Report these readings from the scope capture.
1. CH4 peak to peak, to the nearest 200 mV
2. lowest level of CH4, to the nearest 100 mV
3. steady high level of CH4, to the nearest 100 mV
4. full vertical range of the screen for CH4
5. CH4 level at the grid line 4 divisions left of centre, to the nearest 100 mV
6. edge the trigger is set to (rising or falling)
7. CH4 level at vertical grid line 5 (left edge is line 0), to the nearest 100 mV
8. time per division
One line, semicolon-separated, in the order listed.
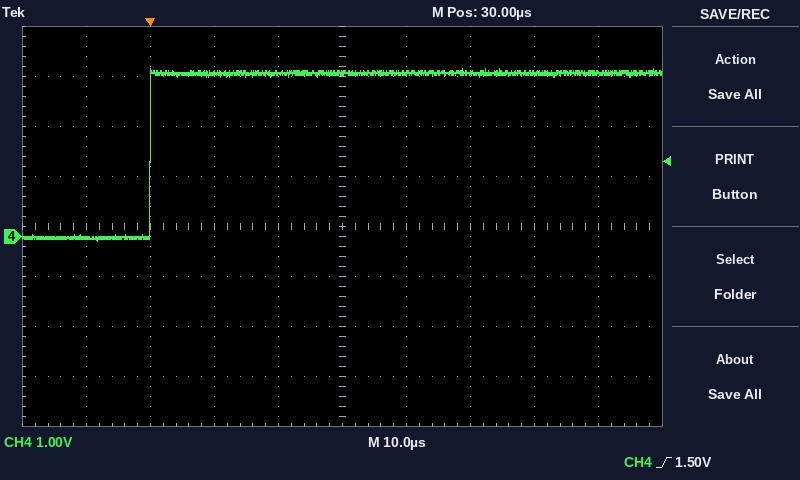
3.4 V; -100 mV; 3.3 V; 8 V; 0.0 V; rising; 3.3 V; 10 µs
